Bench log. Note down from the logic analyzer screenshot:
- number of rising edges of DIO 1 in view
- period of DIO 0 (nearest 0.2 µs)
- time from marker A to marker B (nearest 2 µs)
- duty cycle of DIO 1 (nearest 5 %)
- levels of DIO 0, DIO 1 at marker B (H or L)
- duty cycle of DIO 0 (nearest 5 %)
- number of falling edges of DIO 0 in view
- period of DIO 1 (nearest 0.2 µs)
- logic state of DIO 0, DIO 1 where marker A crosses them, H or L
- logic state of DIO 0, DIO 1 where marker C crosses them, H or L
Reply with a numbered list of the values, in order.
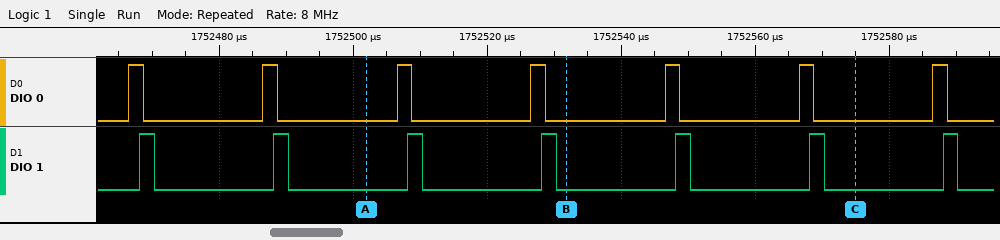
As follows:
1. 7
2. 20 µs
3. 30 µs
4. 10 %
5. DIO 0=L, DIO 1=L
6. 10 %
7. 7
8. 20 µs
9. DIO 0=L, DIO 1=L
10. DIO 0=L, DIO 1=L
